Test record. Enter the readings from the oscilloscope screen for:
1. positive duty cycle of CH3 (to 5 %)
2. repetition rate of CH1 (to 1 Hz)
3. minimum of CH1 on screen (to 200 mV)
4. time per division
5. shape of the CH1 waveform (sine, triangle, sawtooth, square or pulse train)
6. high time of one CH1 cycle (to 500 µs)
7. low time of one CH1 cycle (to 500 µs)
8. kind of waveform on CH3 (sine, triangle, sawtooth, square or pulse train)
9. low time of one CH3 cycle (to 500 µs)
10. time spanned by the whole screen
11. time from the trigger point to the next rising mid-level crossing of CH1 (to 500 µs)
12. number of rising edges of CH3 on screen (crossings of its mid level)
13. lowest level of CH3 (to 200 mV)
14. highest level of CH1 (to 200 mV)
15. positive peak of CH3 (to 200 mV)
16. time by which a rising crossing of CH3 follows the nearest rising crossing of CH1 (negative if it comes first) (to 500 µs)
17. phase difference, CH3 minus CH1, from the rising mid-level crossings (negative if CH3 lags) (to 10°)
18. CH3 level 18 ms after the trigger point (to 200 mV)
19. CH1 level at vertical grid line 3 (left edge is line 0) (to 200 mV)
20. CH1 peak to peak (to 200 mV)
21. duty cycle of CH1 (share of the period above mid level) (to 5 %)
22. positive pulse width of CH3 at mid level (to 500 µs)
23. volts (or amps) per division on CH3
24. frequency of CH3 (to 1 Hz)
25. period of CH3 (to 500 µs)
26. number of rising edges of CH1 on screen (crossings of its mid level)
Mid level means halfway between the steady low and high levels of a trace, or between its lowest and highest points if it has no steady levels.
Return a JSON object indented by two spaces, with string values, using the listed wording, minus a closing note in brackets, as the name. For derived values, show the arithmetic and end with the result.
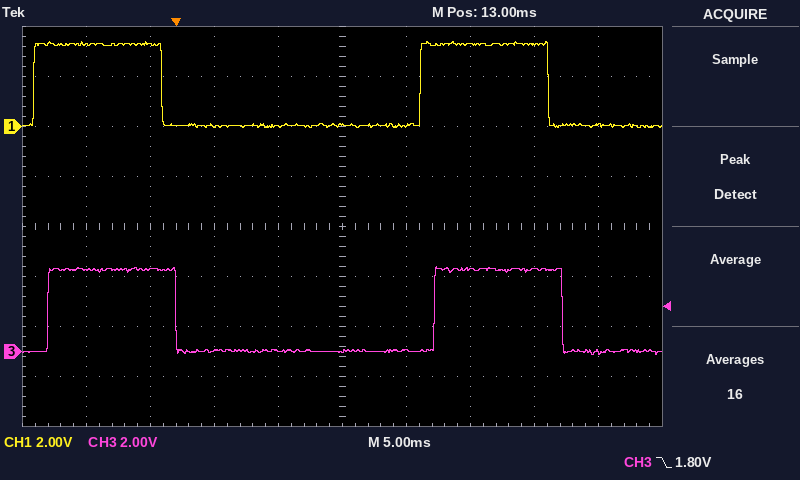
{
  "positive duty cycle of CH3": "10.0 ms / 30.0 ms ≈ 33.3 %, so 35 % to the nearest 5 %",
  "repetition rate of CH1": "1 / 30.0 ms ≈ 33 Hz",
  "minimum of CH1 on screen": "0.0 V",
  "time per division": "5 ms",
  "shape of the CH1 waveform": "pulse train",
  "high time of one CH1 cycle": "10.0 ms",
  "low time of one CH1 cycle": "20.0 ms",
  "kind of waveform on CH3": "pulse train",
  "low time of one CH3 cycle": "20.0 ms",
  "time spanned by the whole screen": "50 ms",
  "time from the trigger point to the next rising mid-level crossing of CH1": "19.0 ms",
  "number of rising edges of CH3 on screen": "2",
  "lowest level of CH3": "-200 mV",
  "highest level of CH1": "3.4 V",
  "positive peak of CH3": "3.4 V",
  "time by which a rising crossing of CH3 follows the nearest rising crossing of CH1 (negative if it comes first)": "+1.0 ms",
  "phase difference, CH3 minus CH1, from the rising mid-level crossings (negative if CH3 lags)": "−360° × (+1.0 ms) / 30.0 ms ≈ -12.0°, so -10° to the nearest 10°",
  "CH3 level 18 ms after the trigger point": "0.0 V",
  "CH1 level at vertical grid line 3 (left edge is line 0)": "0.0 V",
  "CH1 peak to peak": "3.4 V − (0.0 V) = 3.4 V",
  "duty cycle of CH1 (share of the period above mid level)": "10.0 ms / 30.0 ms ≈ 33.3 %, so 35 % to the nearest 5 %",
  "positive pulse width of CH3 at mid level": "10.0 ms",
  "volts (or amps) per division on CH3": "2 V",
  "frequency of CH3": "1 / 30.0 ms ≈ 33 Hz",
  "period of CH3": "30.0 ms",
  "number of rising edges of CH1 on screen": "2"
}
